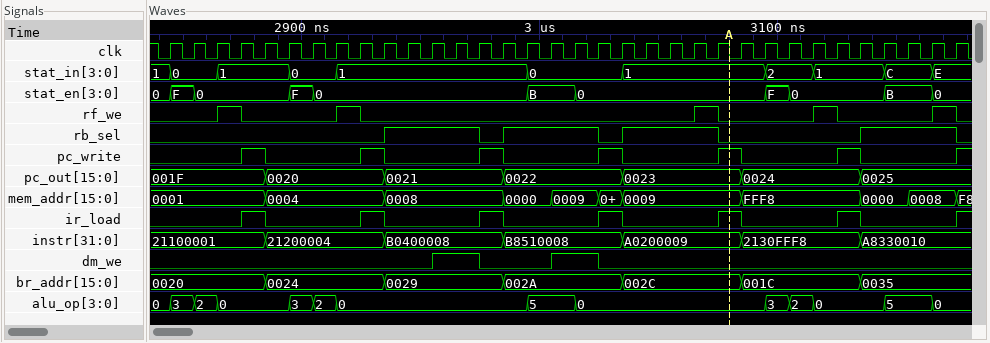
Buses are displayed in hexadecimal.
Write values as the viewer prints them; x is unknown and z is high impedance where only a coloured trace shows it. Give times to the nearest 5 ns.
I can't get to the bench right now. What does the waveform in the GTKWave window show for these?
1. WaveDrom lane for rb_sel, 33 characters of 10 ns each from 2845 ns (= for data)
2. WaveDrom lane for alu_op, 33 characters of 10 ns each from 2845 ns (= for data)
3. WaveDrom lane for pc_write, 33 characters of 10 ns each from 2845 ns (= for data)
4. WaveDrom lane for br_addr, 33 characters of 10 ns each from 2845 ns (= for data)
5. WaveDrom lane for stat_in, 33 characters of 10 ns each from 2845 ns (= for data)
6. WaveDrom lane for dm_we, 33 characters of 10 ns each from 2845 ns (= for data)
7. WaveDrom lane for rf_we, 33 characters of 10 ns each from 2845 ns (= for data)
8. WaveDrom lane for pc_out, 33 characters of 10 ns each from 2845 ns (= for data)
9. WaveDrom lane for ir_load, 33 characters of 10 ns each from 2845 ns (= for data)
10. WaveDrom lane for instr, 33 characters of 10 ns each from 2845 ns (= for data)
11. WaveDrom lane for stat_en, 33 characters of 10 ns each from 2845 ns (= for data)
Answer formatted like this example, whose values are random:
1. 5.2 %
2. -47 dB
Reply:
1. {name: 'rb_sel', wave: '0........1...01...01...0.....1...'}
2. {name: 'alu_op', wave: '===..===.......=.=.......===..=.=', data: '3 2 0 3 2 0 5 0 3 2 0 5 0'}
3. {name: 'pc_write', wave: '0..10...10...10...10...10...10...'}
4. {name: 'br_addr', wave: '=...=....=....=....=....=....=...', data: '0020 0024 0029 002A 002C 001C 0035'}
5. {name: 'stat_in', wave: '=.=..=.=.......=...=.....=.=..=.=', data: '0 1 0 1 0 1 2 1 C E'}
6. {name: 'dm_we', wave: '0..........1.0..1.0..............'}
7. {name: 'rf_we', wave: '0.10...10.............10...10...1'}
8. {name: 'pc_out', wave: '=...=....=....=....=....=....=...', data: '001F 0020 0021 0022 0023 0024 0025'}
9. {name: 'ir_load', wave: '0..10...10...10...10...10...10...'}
10. {name: 'instr', wave: '=...=....=....=....=....=....=...', data: '21100001 21200004 B0400008 B8510008 A0200009 2130FFF8 A8330010'}
11. {name: 'stat_en', wave: '==...==........=.=.......==...=.=', data: 'F 0 F 0 B 0 F 0 B 0'}
